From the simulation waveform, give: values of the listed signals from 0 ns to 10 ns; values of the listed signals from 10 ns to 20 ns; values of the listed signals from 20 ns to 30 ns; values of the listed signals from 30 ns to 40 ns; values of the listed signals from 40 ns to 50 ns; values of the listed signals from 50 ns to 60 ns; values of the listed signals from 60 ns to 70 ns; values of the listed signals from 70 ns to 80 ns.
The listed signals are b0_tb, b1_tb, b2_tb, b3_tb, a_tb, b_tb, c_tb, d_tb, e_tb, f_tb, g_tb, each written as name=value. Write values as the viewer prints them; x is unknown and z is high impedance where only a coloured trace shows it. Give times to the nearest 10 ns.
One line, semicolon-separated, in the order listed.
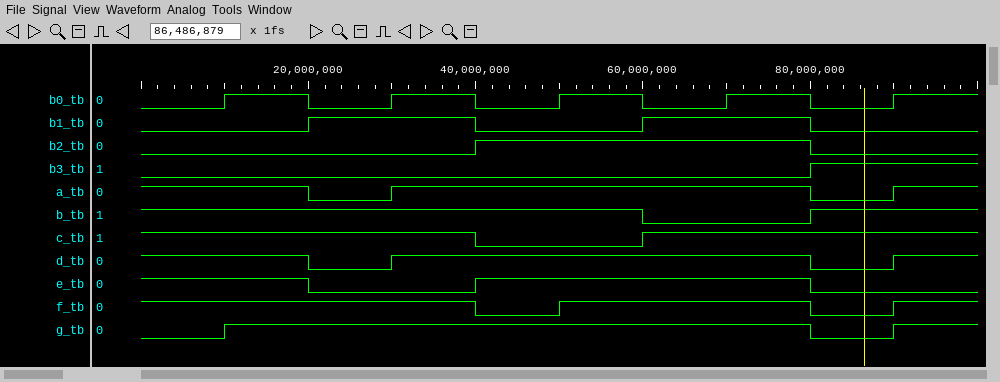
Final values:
b0_tb=0, b1_tb=0, b2_tb=0, b3_tb=0, a_tb=1, b_tb=1, c_tb=1, d_tb=1, e_tb=1, f_tb=1, g_tb=0; b0_tb=1, b1_tb=0, b2_tb=0, b3_tb=0, a_tb=1, b_tb=1, c_tb=1, d_tb=1, e_tb=1, f_tb=1, g_tb=1; b0_tb=0, b1_tb=1, b2_tb=0, b3_tb=0, a_tb=0, b_tb=1, c_tb=1, d_tb=0, e_tb=0, f_tb=1, g_tb=1; b0_tb=1, b1_tb=1, b2_tb=0, b3_tb=0, a_tb=1, b_tb=1, c_tb=1, d_tb=1, e_tb=0, f_tb=1, g_tb=1; b0_tb=0, b1_tb=0, b2_tb=1, b3_tb=0, a_tb=1, b_tb=1, c_tb=0, d_tb=1, e_tb=1, f_tb=0, g_tb=1; b0_tb=1, b1_tb=0, b2_tb=1, b3_tb=0, a_tb=1, b_tb=1, c_tb=0, d_tb=1, e_tb=1, f_tb=1, g_tb=1; b0_tb=0, b1_tb=1, b2_tb=1, b3_tb=0, a_tb=1, b_tb=0, c_tb=1, d_tb=1, e_tb=1, f_tb=1, g_tb=1; b0_tb=1, b1_tb=1, b2_tb=1, b3_tb=0, a_tb=1, b_tb=0, c_tb=1, d_tb=1, e_tb=1, f_tb=1, g_tb=1
